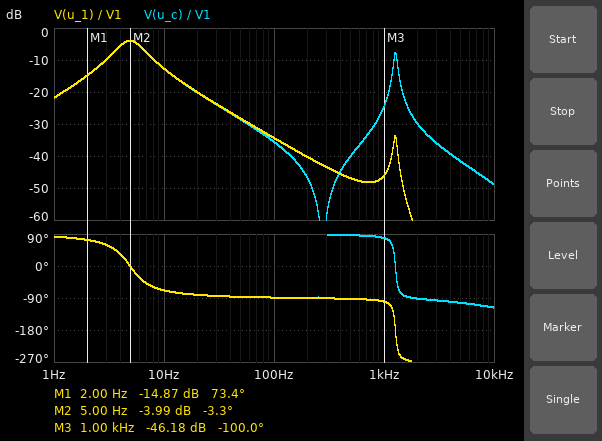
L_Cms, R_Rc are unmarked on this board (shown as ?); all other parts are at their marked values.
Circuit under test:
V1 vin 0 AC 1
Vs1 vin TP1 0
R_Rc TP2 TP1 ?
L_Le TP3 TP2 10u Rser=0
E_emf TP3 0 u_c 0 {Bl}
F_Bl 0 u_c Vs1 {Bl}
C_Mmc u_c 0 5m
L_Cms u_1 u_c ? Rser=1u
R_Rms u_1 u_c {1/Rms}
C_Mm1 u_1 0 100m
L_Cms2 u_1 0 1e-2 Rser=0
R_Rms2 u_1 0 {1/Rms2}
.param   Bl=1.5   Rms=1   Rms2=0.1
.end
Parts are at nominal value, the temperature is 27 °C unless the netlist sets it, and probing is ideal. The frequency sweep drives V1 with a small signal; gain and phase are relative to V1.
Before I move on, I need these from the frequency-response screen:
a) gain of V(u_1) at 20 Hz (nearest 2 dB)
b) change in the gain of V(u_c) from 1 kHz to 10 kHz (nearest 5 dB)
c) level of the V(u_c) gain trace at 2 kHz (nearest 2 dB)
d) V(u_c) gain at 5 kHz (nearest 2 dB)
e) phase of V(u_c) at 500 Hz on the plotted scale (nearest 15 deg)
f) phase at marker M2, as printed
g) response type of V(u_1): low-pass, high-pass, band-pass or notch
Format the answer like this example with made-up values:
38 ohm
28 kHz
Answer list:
-20 dB
-25 dB
-30 dB
-42 dB
90 deg
-3.3 deg
band-pass
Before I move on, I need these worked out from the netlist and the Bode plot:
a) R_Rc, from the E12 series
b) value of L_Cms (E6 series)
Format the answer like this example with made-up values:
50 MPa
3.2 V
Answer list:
1.2 Ω
3.3 µH
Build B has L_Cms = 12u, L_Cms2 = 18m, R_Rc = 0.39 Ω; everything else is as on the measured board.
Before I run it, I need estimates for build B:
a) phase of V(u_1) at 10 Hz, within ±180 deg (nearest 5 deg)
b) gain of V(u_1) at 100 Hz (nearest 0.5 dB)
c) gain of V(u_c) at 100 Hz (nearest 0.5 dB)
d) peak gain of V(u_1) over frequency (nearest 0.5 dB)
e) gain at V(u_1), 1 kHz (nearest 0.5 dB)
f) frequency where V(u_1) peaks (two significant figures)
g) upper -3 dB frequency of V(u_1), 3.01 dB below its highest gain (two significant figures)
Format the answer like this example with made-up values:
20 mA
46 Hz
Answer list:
-45 deg
-24.5 dB
-30.0 dB
-3.5 dB
-47.0 dB
3.7 Hz
10 Hz
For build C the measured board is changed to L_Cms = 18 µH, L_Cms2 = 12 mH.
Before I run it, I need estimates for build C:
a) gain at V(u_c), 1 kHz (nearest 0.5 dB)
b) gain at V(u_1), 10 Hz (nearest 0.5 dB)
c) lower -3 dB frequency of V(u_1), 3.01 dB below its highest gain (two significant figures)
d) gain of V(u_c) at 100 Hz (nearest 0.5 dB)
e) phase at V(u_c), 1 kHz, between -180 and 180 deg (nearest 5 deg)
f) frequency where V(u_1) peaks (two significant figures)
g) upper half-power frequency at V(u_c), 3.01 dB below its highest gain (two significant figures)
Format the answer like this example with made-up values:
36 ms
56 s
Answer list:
-25.0 dB
-13.0 dB
3.2 Hz
-45.0 dB
-85 deg
4.5 Hz
6.2 Hz
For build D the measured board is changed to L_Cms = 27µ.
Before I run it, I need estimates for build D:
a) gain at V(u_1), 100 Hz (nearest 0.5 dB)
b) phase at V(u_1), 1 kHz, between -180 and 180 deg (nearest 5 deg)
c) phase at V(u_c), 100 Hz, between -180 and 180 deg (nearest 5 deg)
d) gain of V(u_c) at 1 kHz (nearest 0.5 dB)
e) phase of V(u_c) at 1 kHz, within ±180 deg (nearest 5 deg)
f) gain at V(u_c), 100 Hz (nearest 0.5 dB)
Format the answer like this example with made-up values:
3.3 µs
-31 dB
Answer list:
-34.0 dB
105 deg
70 deg
-26.0 dB
-85 deg
-57.5 dB
